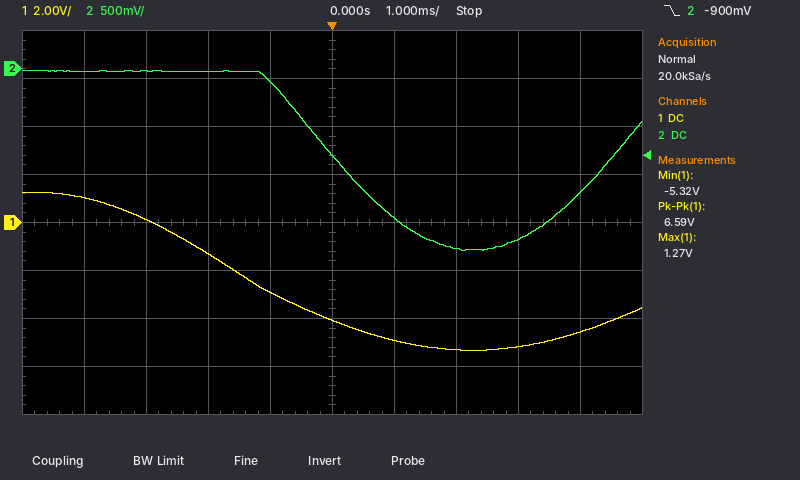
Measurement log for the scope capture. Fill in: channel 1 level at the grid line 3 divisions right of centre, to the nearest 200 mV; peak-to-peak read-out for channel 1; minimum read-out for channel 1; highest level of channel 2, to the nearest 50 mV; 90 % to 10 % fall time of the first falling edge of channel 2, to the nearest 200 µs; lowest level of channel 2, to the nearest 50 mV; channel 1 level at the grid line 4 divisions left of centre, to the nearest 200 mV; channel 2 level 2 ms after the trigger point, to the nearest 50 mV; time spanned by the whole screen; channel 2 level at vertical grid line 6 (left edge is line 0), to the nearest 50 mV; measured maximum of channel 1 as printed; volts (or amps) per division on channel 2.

-5.2 V
6.59 V
-5.32 V
0 mV
2.2 ms
-1.90 V
1.0 V
-1.85 V
10 ms
-1.55 V
1.27 V
500 mV
